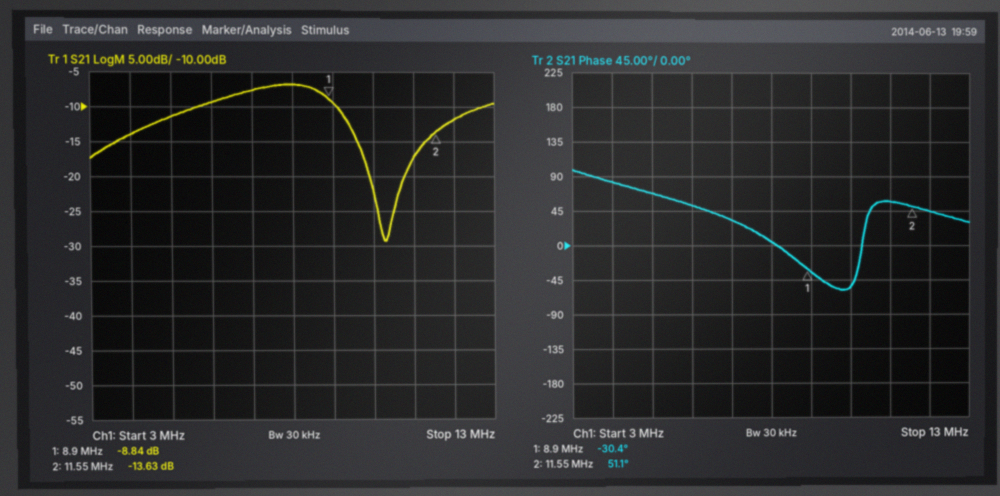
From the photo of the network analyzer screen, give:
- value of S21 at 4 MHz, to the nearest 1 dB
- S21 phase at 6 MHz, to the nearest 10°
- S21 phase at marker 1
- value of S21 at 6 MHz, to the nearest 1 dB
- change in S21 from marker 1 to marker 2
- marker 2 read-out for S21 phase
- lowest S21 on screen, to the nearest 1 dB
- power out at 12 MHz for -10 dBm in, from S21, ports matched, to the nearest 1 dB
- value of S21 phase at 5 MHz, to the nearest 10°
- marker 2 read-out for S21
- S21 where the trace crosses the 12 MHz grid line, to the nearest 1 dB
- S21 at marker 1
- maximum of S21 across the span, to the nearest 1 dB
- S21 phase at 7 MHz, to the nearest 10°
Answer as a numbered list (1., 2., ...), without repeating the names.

1. -14 dB
2. 50°
3. -30.4°
4. -9 dB
5. -4.79 dB
6. 51.1°
7. -29 dB
8. -22 dBm
9. 70°
10. -13.63 dB
11. -12 dB
12. -8.84 dB
13. -7 dB
14. 30°
